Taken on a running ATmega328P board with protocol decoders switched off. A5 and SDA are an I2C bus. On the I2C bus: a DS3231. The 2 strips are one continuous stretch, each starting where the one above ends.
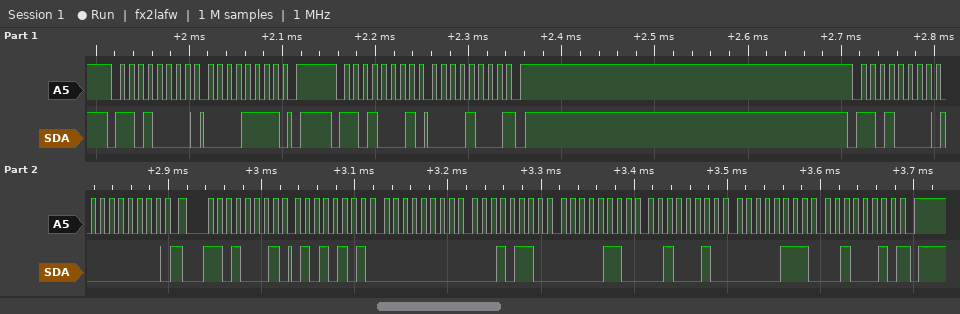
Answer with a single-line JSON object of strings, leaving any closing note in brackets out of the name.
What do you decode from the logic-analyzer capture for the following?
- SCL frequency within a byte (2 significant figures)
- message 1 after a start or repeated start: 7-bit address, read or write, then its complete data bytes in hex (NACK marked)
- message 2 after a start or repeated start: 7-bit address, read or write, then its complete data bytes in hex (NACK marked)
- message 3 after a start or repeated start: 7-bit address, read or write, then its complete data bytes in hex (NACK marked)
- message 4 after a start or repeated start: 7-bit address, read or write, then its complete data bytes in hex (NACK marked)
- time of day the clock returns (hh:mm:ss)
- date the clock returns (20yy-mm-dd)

{"SCL frequency within a byte": "100 kHz", "message 1 after a start or repeated start: 7-bit address, read or write, then its complete data bytes in hex": "0x68 write: 0F", "message 2 after a start or repeated start: 7-bit address, read or write, then its complete data bytes in hex": "0x68 read: 08 NACK", "message 3 after a start or repeated start: 7-bit address, read or write, then its complete data bytes in hex": "0x68 write: 00", "message 4 after a start or repeated start: 7-bit address, read or write, then its complete data bytes in hex": "0x68 read: 55 00 16 06 22 07 22 NACK", "time of day the clock returns": "16:00:55", "date the clock returns": "2022-07-22"}
